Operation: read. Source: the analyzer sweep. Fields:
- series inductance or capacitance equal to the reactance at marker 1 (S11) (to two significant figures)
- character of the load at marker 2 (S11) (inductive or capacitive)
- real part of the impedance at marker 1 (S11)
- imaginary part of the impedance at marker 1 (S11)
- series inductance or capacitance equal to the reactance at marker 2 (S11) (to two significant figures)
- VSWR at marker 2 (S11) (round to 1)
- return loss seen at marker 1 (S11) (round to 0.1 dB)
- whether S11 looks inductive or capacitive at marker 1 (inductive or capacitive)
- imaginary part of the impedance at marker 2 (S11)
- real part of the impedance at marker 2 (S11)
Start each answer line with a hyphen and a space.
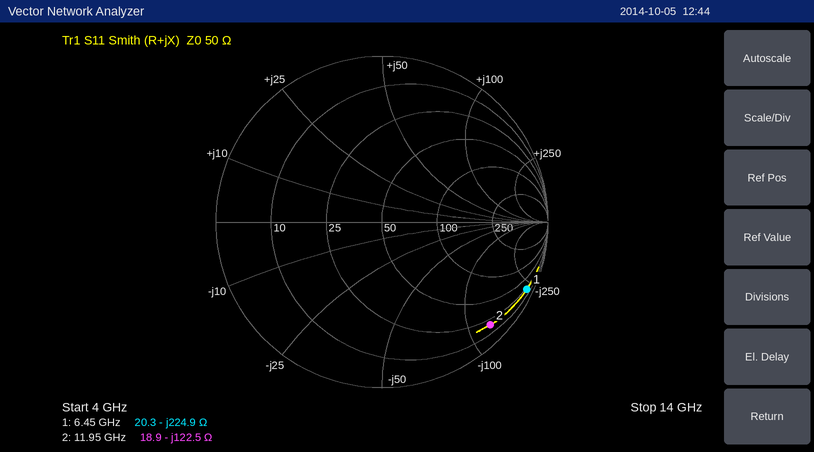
- 110 fF
- capacitive
- 20.3 Ω
- -224.9 Ω
- 110 fF
- 19
- 0.3 dB
- capacitive
- -122.5 Ω
- 18.9 Ω
